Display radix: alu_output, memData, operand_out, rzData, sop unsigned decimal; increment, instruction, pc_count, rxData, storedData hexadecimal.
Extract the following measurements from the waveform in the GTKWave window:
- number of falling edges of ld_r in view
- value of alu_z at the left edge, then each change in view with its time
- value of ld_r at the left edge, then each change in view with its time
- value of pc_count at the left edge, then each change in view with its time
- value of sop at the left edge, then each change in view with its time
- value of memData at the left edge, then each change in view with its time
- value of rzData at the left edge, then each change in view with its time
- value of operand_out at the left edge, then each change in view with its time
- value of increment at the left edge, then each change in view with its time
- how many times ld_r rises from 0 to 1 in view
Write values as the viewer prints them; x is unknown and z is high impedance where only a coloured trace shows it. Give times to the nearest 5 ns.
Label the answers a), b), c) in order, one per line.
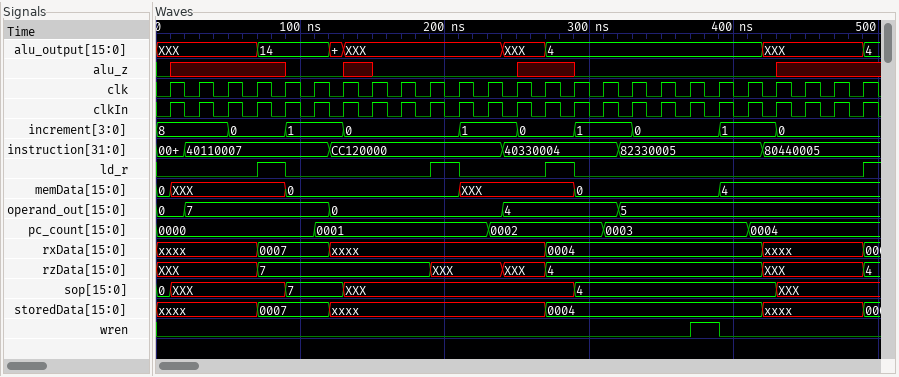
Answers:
a) 3
b) 0, x at 10 ns, 0 at 90 ns, x at 130 ns, 0 at 150 ns, x at 250 ns, 0 at 290 ns, x at 430 ns
c) 0, 1 at 70 ns, 0 at 90 ns, 1 at 190 ns, 0 at 210 ns, 1 at 270 ns, 0 at 290 ns, 1 at 490 ns
d) 0000, 0001 at 110 ns, 0002 at 230 ns, 0003 at 310 ns, 0004 at 410 ns
e) 0, XXX at 10 ns, 7 at 90 ns, XXX at 130 ns, 4 at 290 ns, XXX at 430 ns
f) 0, XXX at 10 ns, 0 at 90 ns, XXX at 210 ns, 0 at 290 ns, 4 at 390 ns
g) XXX, 7 at 70 ns, XXX at 190 ns, XXX at 240 ns, 4 at 270 ns, XXX at 420 ns, 4 at 490 ns
h) 0, 7 at 20 ns, 0 at 120 ns, 4 at 240 ns, 5 at 320 ns
i) 8, 0 at 50 ns, 1 at 90 ns, 0 at 130 ns, 1 at 210 ns, 0 at 250 ns, 1 at 290 ns, 0 at 330 ns, 1 at 390 ns, 0 at 430 ns
j) 4
